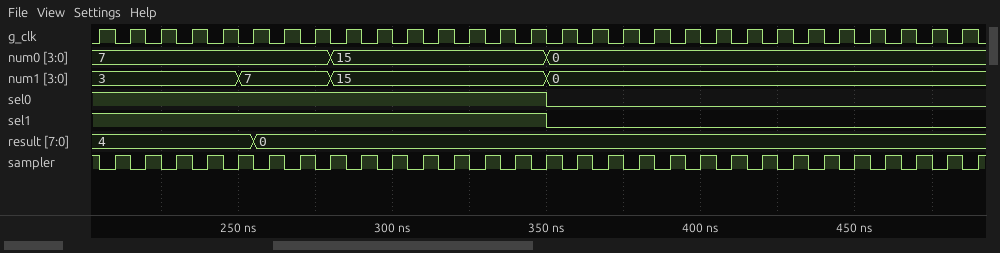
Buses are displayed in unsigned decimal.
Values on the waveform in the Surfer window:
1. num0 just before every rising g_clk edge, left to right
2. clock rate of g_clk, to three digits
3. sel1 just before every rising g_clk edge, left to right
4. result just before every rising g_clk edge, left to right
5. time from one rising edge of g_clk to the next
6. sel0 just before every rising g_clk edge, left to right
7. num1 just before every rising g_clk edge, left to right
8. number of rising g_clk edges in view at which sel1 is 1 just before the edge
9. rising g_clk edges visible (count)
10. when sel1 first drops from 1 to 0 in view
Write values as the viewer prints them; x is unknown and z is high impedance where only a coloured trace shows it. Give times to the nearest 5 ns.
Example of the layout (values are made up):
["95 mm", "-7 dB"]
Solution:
["7, 7, 7, 7, 7, 7, 7, 7, 15, 15, 15, 15, 15, 15, 15, 0, 0, 0, 0, 0, 0, 0, 0, 0, 0, 0, 0, 0, 0", "100 MHz", "1 1 1 1 1 1 1 1 1 1 1 1 1 1 1 0 0 0 0 0 0 0 0 0 0 0 0 0 0", "4, 4, 4, 4, 4, 4, 0, 0, 0, 0, 0, 0, 0, 0, 0, 0, 0, 0, 0, 0, 0, 0, 0, 0, 0, 0, 0, 0, 0", "10 ns", "1 1 1 1 1 1 1 1 1 1 1 1 1 1 1 0 0 0 0 0 0 0 0 0 0 0 0 0 0", "3, 3, 3, 3, 3, 7, 7, 7, 15, 15, 15, 15, 15, 15, 15, 0, 0, 0, 0, 0, 0, 0, 0, 0, 0, 0, 0, 0, 0", "15", "29", "350 ns"]
